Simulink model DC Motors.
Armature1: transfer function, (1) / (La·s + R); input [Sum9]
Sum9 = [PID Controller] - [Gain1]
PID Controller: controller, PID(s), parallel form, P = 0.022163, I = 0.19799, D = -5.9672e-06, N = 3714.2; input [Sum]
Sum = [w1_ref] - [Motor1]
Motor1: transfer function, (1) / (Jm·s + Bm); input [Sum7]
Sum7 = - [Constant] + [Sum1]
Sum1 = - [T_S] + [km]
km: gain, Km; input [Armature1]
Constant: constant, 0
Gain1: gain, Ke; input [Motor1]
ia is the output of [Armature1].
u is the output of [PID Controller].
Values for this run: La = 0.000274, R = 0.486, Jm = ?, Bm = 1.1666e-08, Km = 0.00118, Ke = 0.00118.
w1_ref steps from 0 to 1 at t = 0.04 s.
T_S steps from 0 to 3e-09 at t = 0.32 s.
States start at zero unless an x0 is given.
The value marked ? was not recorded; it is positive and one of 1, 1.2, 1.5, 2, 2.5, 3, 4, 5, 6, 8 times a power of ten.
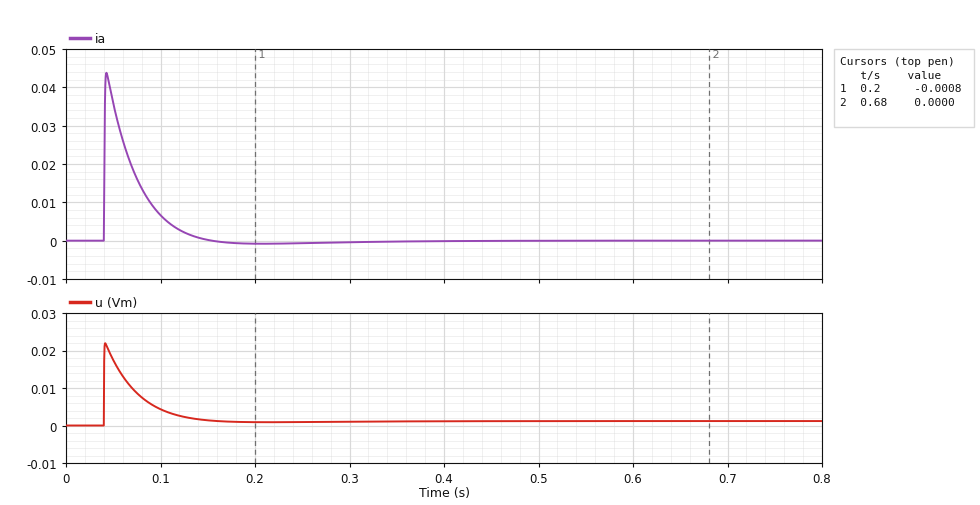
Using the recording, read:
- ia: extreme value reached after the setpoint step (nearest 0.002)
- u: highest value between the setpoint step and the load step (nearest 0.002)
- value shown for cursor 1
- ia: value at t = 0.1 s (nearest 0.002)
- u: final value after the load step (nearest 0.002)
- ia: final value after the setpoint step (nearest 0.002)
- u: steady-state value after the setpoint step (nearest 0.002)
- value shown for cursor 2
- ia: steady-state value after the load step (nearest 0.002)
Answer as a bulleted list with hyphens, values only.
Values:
- 0.044
- 0.022
- -0.0008
- 0.006
- 0.002
- 0.000
- 0.002
- 0.0000
- 0.000
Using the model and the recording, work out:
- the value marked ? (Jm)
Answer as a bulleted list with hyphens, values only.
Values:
- 1.5e-06
